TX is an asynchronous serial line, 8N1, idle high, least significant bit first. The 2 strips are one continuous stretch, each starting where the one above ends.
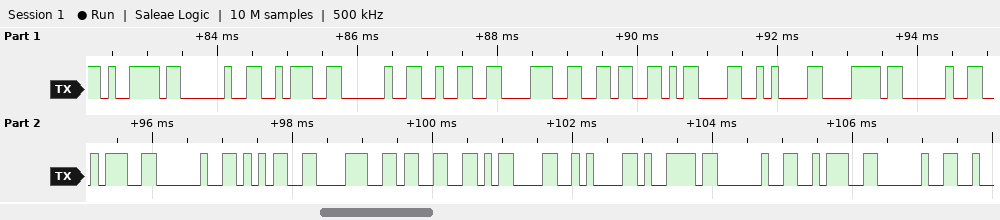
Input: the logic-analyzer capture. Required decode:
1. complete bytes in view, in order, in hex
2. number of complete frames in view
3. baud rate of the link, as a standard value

79 20 3A 20 32 38 36 0D 0A 78 20 3A 20 35 38 33 0D 0A 79 20 3A 20
22
9600 baud
